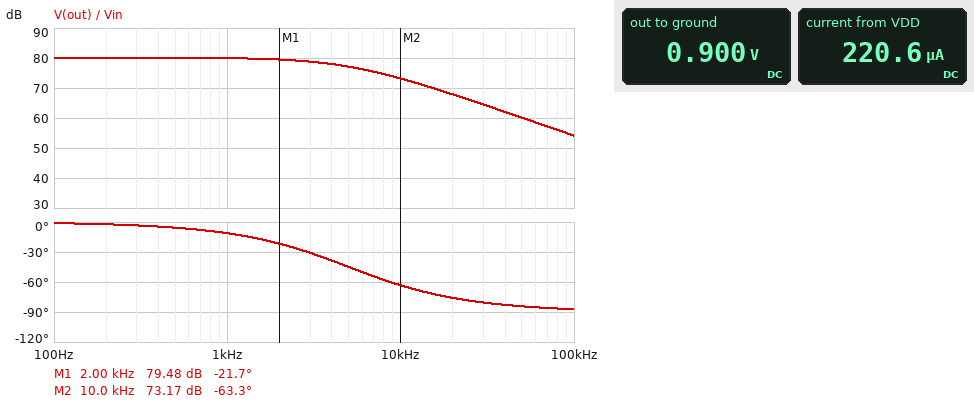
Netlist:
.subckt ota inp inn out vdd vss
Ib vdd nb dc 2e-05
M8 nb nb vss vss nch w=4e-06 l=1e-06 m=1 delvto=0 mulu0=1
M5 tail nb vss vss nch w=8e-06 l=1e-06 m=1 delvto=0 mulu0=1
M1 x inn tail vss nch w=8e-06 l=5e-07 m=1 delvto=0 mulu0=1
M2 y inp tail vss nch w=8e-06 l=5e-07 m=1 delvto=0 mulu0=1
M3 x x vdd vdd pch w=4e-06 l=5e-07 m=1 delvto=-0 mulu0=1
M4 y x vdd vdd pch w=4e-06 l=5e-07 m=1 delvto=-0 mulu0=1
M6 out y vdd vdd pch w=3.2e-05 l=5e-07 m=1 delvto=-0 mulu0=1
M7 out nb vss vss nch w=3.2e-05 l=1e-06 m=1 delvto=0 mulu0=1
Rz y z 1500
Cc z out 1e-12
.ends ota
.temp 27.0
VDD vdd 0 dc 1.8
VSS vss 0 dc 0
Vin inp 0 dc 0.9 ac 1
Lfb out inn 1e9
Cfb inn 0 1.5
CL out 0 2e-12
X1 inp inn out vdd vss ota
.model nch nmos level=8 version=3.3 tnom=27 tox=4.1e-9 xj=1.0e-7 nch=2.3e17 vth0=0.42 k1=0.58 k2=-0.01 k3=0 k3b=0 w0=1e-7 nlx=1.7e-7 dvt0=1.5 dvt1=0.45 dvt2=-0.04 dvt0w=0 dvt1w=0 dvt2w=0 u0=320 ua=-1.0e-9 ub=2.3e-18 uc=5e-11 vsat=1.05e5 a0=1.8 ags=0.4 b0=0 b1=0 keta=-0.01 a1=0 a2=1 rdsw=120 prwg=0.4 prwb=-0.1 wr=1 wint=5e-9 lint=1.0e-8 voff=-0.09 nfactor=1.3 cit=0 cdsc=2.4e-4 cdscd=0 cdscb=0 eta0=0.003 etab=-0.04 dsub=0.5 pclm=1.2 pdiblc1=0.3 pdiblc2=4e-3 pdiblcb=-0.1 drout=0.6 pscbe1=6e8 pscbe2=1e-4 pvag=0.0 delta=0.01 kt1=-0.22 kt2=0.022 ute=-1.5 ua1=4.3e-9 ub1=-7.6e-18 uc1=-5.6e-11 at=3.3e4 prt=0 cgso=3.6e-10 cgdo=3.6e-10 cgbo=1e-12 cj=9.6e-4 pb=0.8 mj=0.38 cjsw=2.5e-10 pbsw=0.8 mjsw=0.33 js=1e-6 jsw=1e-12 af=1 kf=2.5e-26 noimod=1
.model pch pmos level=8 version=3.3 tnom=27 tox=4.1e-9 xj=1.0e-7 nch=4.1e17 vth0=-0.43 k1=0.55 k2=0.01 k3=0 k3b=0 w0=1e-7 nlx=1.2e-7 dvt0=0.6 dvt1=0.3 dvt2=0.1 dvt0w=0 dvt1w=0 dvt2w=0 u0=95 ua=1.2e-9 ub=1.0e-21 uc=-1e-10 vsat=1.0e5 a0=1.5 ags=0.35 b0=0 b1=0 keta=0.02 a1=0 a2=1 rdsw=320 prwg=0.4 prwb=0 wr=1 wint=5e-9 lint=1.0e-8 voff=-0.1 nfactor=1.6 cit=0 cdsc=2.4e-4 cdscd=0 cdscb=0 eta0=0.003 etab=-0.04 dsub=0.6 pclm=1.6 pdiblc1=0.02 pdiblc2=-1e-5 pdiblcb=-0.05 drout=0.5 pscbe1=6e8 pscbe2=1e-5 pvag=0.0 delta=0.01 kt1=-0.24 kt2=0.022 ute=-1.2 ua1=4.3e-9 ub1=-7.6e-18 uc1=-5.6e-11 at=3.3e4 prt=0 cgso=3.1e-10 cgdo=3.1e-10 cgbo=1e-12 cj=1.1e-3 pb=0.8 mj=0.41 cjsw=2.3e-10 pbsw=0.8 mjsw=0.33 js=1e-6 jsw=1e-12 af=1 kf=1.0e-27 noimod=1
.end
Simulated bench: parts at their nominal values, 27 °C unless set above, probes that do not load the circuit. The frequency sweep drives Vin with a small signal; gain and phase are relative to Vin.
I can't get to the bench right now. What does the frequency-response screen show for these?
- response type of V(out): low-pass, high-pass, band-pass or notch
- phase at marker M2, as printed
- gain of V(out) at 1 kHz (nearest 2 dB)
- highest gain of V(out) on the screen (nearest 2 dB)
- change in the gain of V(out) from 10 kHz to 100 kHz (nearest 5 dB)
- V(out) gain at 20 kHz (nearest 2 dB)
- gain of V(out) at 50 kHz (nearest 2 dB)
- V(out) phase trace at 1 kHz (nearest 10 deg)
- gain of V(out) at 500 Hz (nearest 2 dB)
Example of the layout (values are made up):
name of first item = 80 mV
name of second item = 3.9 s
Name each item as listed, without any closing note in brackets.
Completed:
response type of V(out): low-pass, high-pass, band-pass or notch = low-pass
phase at marker M2, as printed = -63.3 deg
gain of V(out) at 1 kHz = 80 dB
highest gain of V(out) on the screen = 80 dB
change in the gain of V(out) from 10 kHz to 100 kHz = -20 dB
V(out) gain at 20 kHz = 68 dB
gain of V(out) at 50 kHz = 60 dB
V(out) phase trace at 1 kHz = -10 deg
gain of V(out) at 500 Hz = 80 dB
